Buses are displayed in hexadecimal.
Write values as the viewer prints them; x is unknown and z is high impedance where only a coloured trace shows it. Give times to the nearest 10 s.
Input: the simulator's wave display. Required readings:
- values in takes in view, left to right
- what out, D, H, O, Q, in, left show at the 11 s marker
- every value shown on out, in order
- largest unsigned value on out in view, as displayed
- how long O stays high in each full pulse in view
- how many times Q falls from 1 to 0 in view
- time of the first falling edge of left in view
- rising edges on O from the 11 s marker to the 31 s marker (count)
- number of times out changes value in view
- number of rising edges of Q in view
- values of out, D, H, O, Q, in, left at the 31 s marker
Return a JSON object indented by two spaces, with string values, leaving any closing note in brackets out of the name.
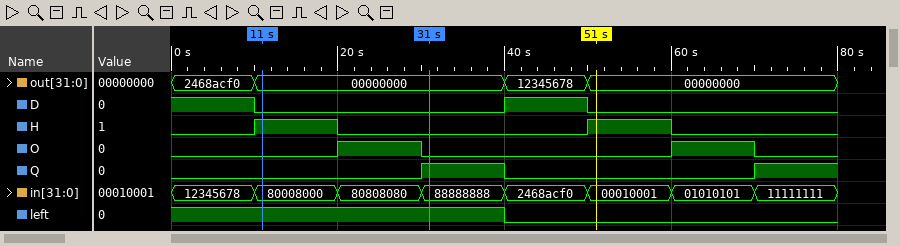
{
  "values in takes in view, left to right": "12345678, 80008000, 80808080, 88888888, 2468acf0, 00010001, 01010101, 11111111",
  "what out, D, H, O, Q, in, left show at the 11 s marker": "out=00000000, D=0, H=1, O=0, Q=0, in=80008000, left=1",
  "every value shown on out, in order": "2468acf0, 00000000, 12345678, 00000000",
  "largest unsigned value on out in view, as displayed": "2468acf0",
  "how long O stays high in each full pulse in view": "10 s, 10 s",
  "how many times Q falls from 1 to 0 in view": "1",
  "time of the first falling edge of left in view": "40 s",
  "rising edges on O from the 11 s marker to the 31 s marker": "1",
  "number of times out changes value in view": "3",
  "number of rising edges of Q in view": "2",
  "values of out, D, H, O, Q, in, left at the 31 s marker": "out=00000000, D=0, H=0, O=0, Q=1, in=88888888, left=1"
}
